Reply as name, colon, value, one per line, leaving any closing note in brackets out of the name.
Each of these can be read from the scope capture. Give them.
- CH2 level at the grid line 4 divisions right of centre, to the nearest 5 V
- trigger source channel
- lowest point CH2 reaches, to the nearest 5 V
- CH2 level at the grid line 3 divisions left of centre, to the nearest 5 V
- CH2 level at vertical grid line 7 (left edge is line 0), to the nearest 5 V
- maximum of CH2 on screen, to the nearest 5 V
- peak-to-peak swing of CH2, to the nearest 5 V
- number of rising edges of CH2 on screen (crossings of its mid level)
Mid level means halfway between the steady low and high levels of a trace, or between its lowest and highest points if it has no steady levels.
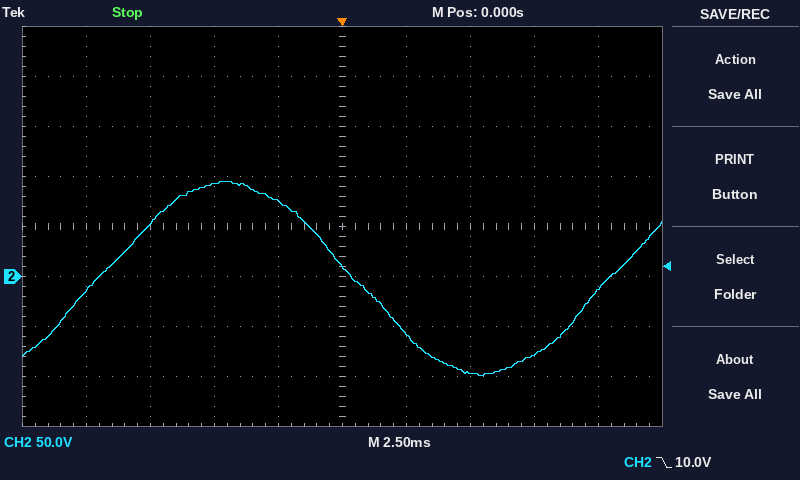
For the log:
CH2 level at the grid line 4 divisions right of centre, to the nearest 5 V: -15 V
trigger source channel: CH2
lowest point CH2 reaches, to the nearest 5 V: -100 V
CH2 level at the grid line 3 divisions left of centre, to the nearest 5 V: 55 V
CH2 level at vertical grid line 7 (left edge is line 0), to the nearest 5 V: -95 V
maximum of CH2 on screen, to the nearest 5 V: 95 V
peak-to-peak swing of CH2, to the nearest 5 V: 195 V
number of rising edges of CH2 on screen: 2
